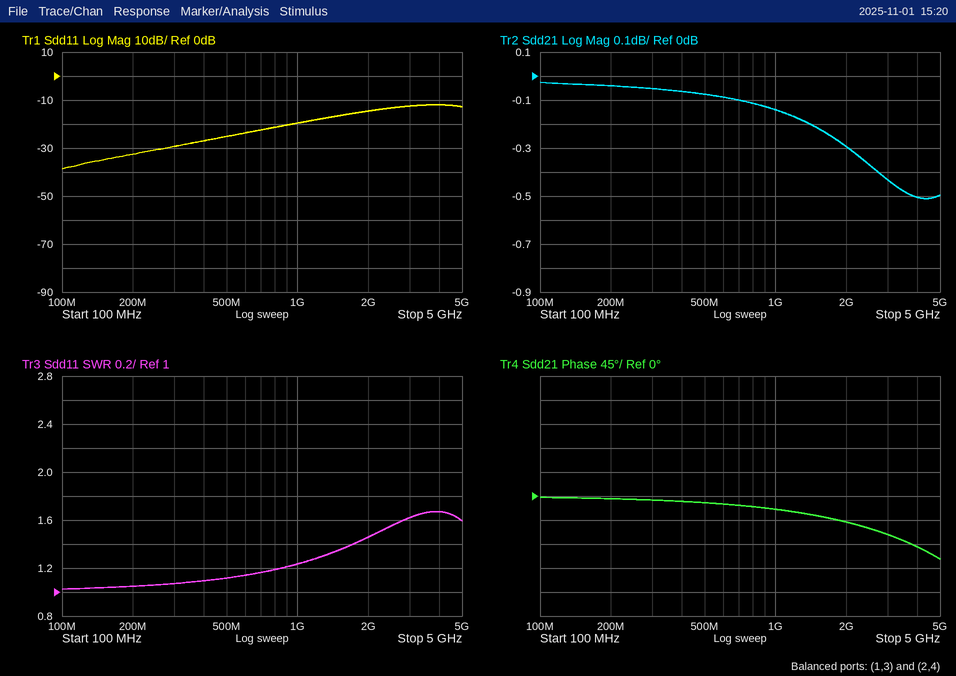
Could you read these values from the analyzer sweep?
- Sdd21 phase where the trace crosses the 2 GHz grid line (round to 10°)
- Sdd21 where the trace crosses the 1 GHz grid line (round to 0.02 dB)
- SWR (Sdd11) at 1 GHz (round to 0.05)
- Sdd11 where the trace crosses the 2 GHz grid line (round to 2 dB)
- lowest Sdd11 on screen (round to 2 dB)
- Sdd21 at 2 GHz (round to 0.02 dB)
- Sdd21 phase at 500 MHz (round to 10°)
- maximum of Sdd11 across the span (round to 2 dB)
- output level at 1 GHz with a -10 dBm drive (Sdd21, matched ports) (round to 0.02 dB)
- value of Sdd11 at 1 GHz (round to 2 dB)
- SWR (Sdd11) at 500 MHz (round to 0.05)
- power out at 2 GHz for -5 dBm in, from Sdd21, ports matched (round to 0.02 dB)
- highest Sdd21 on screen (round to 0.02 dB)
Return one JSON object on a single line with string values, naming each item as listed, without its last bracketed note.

{"Sdd21 phase where the trace crosses the 2 GHz grid line": "-50°", "Sdd21 where the trace crosses the 1 GHz grid line": "-0.14 dB", "SWR (Sdd11) at 1 GHz": "1.25", "Sdd11 where the trace crosses the 2 GHz grid line": "-14 dB", "lowest Sdd11 on screen": "-38 dB", "Sdd21 at 2 GHz": "-0.30 dB", "Sdd21 phase at 500 MHz": "-10°", "maximum of Sdd11 across the span": "-12 dB", "output level at 1 GHz with a -10 dBm drive (Sdd21, matched ports)": "-10.14 dBm", "value of Sdd11 at 1 GHz": "-20 dB", "SWR (Sdd11) at 500 MHz": "1.10", "power out at 2 GHz for -5 dBm in, from Sdd21, ports matched": "-5.30 dBm", "highest Sdd21 on screen": "-0.02 dB"}
